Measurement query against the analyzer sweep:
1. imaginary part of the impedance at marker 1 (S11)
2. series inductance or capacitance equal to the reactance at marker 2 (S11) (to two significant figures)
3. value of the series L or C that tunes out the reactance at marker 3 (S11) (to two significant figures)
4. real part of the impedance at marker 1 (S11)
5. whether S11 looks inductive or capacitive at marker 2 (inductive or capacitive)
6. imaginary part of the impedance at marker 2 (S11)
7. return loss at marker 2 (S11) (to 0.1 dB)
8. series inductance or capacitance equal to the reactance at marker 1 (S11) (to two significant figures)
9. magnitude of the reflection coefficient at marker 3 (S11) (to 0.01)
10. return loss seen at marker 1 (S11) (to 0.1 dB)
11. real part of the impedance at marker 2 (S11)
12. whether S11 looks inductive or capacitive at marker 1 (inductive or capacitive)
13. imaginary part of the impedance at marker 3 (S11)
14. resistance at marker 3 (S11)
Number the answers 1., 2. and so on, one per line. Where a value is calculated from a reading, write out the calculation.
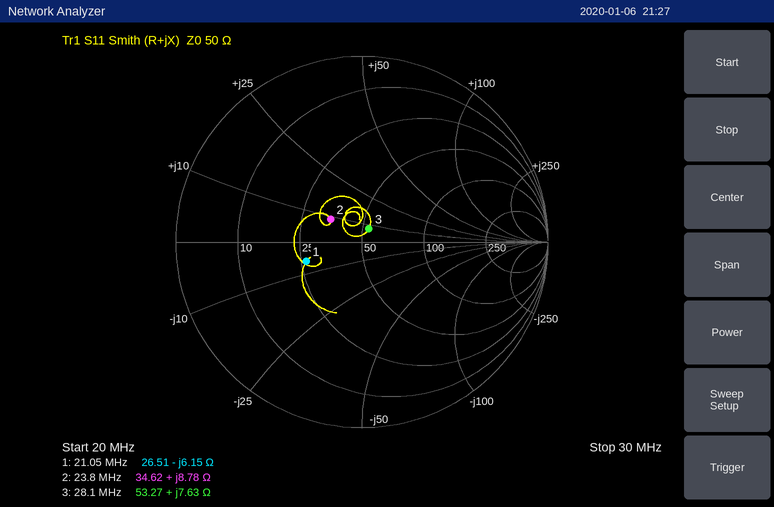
1. -6.15 Ω
2. L = 8.78 Ω/(2π × 23.8 MHz) ≈ 59 nH
3. C = 1/(2π × 28.1 MHz × 7.63 Ω) ≈ 742 pF, so 740 pF to two significant figures
4. 26.51 Ω
5. inductive
6. +8.78 Ω
7. 13.6 dB
8. C = 1/(2π × 21.05 MHz × 6.15 Ω) ≈ 1.2 nF
9. 0.08
10. 10.0 dB
11. 34.62 Ω
12. capacitive
13. +7.63 Ω
14. 53.27 Ω
